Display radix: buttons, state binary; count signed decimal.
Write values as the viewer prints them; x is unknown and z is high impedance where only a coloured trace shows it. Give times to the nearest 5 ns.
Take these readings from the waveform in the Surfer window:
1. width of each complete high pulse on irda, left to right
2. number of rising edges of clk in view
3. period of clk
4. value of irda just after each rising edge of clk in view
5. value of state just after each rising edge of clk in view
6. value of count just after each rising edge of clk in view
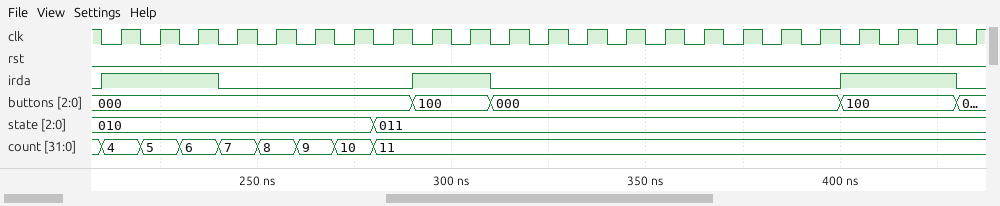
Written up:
30 ns, 20 ns, 30 ns
23
10 ns
1 1 1 0 0 0 0 0 1 1 0 0 0 0 0 0 0 0 0 1 1 1 0
010, 010, 010, 010, 010, 010, 010, 011, 011, 011, 011, 011, 011, 011, 011, 011, 011, 011, 011, 011, 011, 011, 011
4, 5, 6, 7, 8, 9, 10, 11, 11, 11, 11, 11, 11, 11, 11, 11, 11, 11, 11, 11, 11, 11, 11
